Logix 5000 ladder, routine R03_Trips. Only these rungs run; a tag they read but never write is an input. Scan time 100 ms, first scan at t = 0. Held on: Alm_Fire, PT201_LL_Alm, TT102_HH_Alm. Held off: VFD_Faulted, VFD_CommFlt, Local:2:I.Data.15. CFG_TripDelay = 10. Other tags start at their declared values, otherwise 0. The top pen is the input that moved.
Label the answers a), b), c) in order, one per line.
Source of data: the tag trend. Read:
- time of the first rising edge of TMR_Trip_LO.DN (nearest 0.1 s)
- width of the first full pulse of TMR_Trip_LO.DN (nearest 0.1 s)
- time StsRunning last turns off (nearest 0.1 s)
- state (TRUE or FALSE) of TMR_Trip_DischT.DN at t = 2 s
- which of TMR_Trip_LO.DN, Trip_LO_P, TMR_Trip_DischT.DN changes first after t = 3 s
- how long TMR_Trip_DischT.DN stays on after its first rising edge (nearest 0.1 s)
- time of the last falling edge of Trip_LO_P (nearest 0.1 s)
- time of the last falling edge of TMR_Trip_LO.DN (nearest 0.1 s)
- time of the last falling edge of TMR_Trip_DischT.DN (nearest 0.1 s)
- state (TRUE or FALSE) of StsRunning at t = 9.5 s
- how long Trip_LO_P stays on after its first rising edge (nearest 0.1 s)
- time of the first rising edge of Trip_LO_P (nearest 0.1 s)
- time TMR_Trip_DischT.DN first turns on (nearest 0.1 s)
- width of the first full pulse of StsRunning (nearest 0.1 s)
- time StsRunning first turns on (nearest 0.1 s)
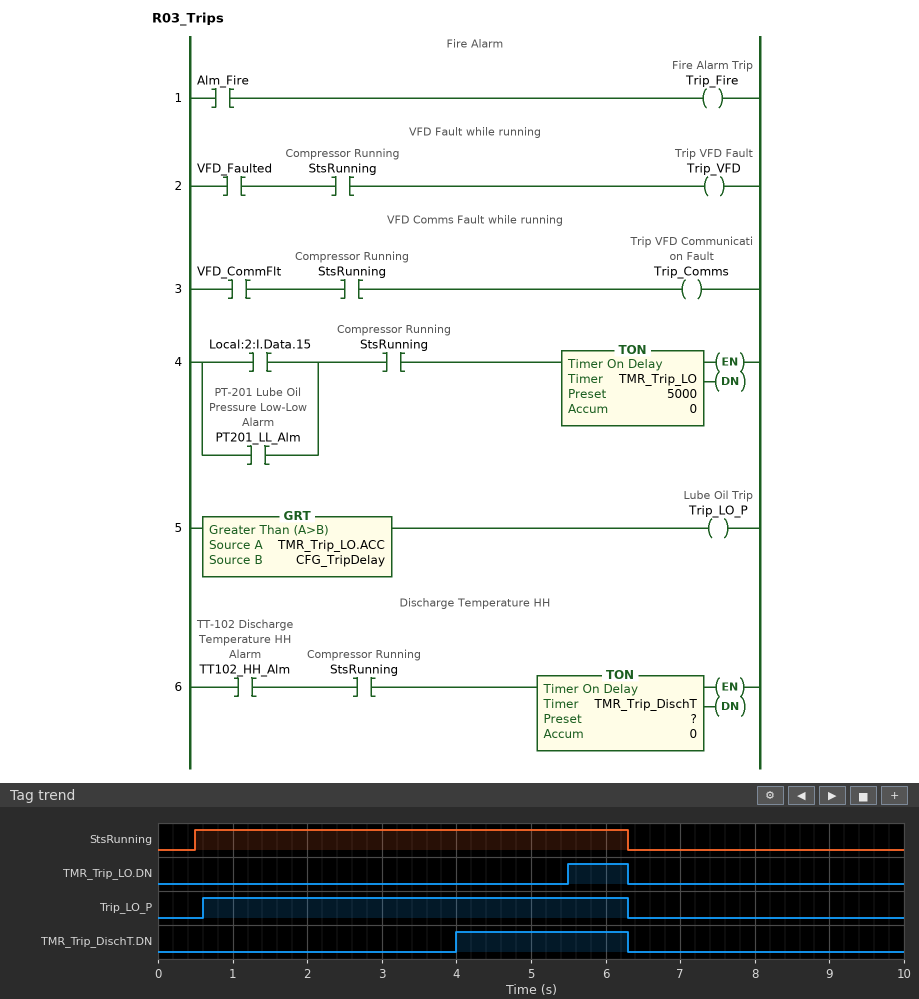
a) 5.5 s
b) 0.8 s
c) 6.3 s
d) FALSE
e) TMR_Trip_DischT.DN
f) 2.3 s
g) 6.3 s
h) 6.3 s
i) 6.3 s
j) FALSE
k) 5.7 s
l) 0.6 s
m) 4.0 s
n) 5.8 s
o) 0.5 s
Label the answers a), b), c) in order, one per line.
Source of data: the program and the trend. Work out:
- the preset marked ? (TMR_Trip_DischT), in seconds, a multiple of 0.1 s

a) 3.5 s
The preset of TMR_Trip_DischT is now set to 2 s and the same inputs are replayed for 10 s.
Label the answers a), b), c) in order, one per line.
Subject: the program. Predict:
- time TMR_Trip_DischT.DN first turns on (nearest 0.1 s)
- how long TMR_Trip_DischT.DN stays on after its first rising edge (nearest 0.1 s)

a) 2.5 s
b) 3.8 s
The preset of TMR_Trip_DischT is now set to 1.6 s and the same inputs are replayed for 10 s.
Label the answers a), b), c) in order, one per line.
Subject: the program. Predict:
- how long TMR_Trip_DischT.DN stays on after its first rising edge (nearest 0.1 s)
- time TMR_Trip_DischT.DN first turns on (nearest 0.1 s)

a) 4.2 s
b) 2.1 s
